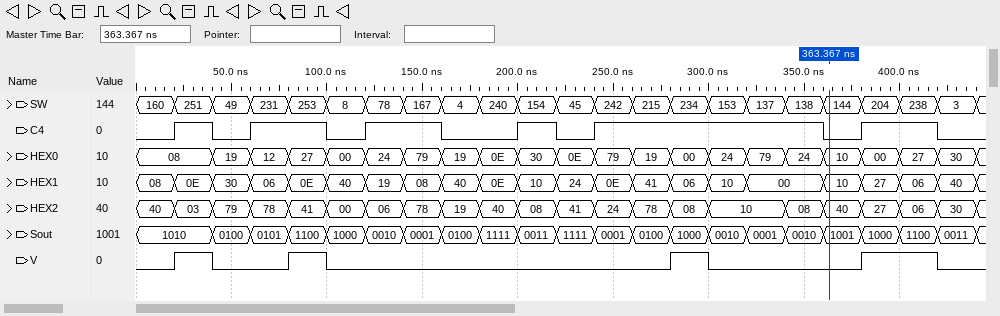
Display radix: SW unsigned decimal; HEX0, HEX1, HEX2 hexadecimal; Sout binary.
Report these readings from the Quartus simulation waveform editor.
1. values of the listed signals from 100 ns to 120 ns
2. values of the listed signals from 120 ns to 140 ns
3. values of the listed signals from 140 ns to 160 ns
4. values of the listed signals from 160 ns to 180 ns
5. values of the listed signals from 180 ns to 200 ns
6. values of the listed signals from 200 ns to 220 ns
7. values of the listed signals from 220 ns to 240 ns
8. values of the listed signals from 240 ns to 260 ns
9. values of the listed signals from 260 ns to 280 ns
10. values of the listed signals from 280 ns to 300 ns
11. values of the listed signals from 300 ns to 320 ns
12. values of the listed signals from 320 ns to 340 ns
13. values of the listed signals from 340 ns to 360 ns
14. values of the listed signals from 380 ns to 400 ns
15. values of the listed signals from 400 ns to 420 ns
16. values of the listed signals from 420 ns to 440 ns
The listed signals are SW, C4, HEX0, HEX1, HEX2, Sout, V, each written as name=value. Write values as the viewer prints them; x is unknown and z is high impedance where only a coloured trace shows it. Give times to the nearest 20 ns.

SW=8, C4=0, HEX0=00, HEX1=40, HEX2=00, Sout=1000, V=0
SW=78, C4=1, HEX0=24, HEX1=19, HEX2=06, Sout=0010, V=0
SW=167, C4=1, HEX0=79, HEX1=08, HEX2=78, Sout=0001, V=0
SW=4, C4=0, HEX0=19, HEX1=40, HEX2=19, Sout=0100, V=0
SW=240, C4=0, HEX0=0E, HEX1=0E, HEX2=40, Sout=1111, V=0
SW=154, C4=1, HEX0=30, HEX1=10, HEX2=08, Sout=0011, V=0
SW=45, C4=0, HEX0=0E, HEX1=24, HEX2=41, Sout=1111, V=0
SW=242, C4=1, HEX0=79, HEX1=0E, HEX2=24, Sout=0001, V=0
SW=215, C4=1, HEX0=19, HEX1=41, HEX2=78, Sout=0100, V=0
SW=234, C4=1, HEX0=00, HEX1=06, HEX2=08, Sout=1000, V=1
SW=153, C4=1, HEX0=24, HEX1=10, HEX2=10, Sout=0010, V=0
SW=137, C4=1, HEX0=79, HEX1=00, HEX2=10, Sout=0001, V=0
SW=138, C4=1, HEX0=24, HEX1=00, HEX2=08, Sout=0010, V=0
SW=204, C4=1, HEX0=00, HEX1=27, HEX2=27, Sout=1000, V=1
SW=238, C4=1, HEX0=27, HEX1=06, HEX2=06, Sout=1100, V=1
SW=3, C4=0, HEX0=30, HEX1=40, HEX2=30, Sout=0011, V=0
